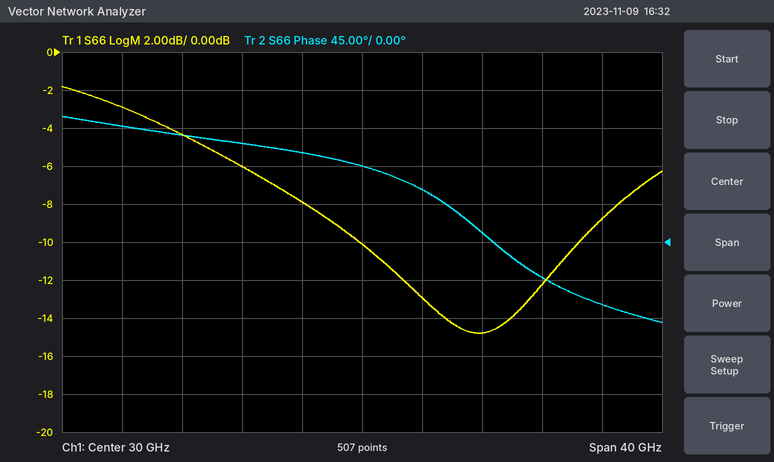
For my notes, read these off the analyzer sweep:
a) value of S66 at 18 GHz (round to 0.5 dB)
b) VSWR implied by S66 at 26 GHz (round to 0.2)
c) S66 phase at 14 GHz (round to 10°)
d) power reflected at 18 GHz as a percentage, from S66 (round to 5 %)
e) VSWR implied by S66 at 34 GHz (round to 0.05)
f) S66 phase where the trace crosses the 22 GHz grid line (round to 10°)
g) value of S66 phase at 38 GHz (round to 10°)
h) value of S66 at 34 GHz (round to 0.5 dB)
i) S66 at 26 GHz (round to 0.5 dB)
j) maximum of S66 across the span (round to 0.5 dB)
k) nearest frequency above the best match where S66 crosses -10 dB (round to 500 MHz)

-4.5 dB
2.4
140°
35 %
1.60
120°
10°
-13.0 dB
-8.0 dB
-2.0 dB
44.5 GHz
